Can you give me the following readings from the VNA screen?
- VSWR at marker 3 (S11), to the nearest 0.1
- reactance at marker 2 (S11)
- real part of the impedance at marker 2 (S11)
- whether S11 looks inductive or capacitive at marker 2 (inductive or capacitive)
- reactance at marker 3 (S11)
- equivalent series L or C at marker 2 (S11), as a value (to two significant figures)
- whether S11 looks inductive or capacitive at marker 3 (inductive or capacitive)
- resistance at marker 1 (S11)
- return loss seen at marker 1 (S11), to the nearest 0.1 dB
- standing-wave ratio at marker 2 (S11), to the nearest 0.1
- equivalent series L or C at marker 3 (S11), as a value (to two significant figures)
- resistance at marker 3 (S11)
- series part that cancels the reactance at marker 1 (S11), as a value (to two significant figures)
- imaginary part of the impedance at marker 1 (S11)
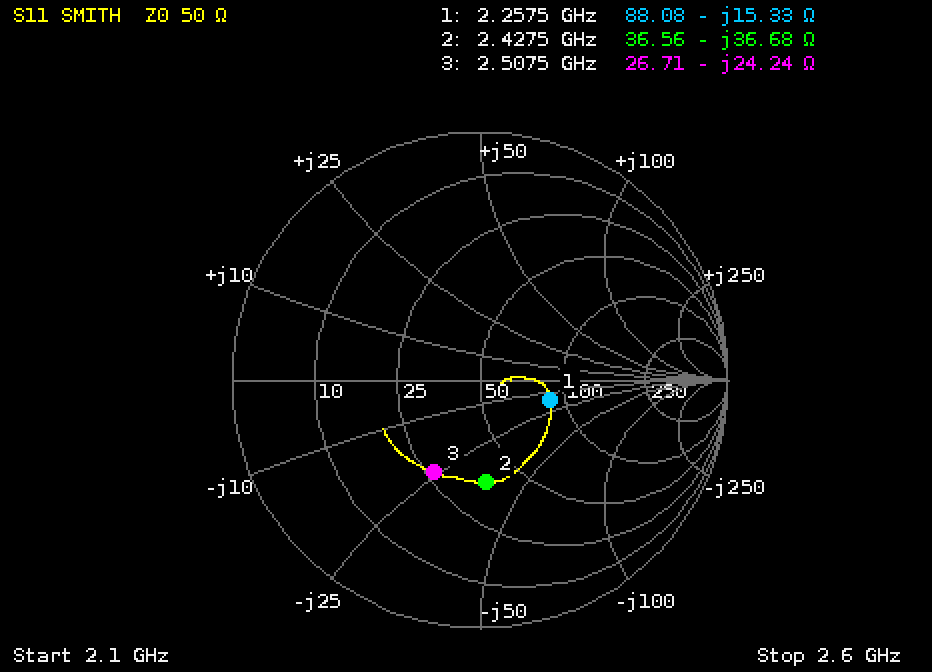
2.4
-36.68 Ω
36.56 Ω
capacitive
-24.24 Ω
1.8 pF
capacitive
88.08 Ω
10.6 dB
2.4
2.6 pF
26.71 Ω
1.1 nH
-15.33 Ω
